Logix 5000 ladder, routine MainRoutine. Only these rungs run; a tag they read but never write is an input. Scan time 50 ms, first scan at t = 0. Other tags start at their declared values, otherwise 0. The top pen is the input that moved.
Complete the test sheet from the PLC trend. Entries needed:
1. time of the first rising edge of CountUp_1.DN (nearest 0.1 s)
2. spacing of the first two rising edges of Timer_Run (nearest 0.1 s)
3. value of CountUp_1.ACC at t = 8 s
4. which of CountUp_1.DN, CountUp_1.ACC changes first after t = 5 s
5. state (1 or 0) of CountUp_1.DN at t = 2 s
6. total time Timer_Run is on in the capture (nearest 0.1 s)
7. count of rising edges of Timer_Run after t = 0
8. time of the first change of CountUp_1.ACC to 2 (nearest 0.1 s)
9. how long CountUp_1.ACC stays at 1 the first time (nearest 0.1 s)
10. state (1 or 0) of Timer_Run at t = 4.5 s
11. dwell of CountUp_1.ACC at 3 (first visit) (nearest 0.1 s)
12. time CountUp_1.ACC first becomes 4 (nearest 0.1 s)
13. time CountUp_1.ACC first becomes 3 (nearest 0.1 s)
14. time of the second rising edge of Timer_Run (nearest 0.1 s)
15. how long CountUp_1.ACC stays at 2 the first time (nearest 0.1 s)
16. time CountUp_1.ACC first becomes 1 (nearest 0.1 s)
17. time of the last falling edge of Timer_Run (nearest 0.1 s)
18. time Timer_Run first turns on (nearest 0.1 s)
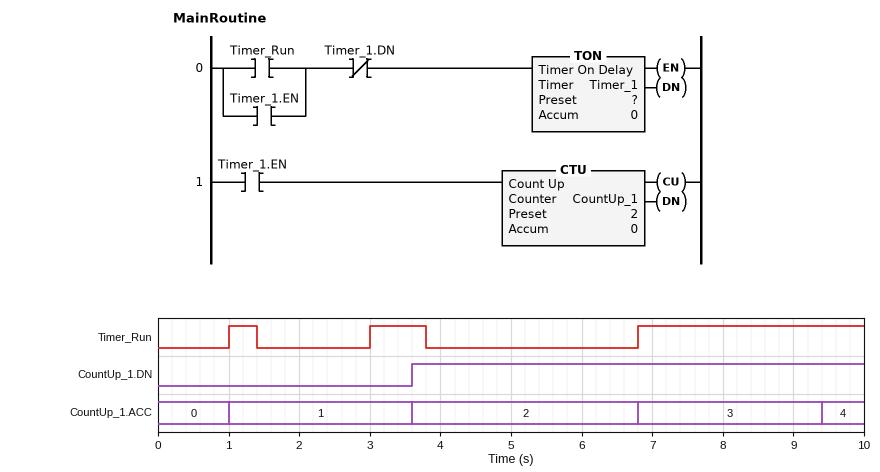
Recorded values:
3.6 s
2.0 s
3
CountUp_1.ACC
0
4.4 s
3
3.6 s
2.6 s
0
2.6 s
9.4 s
6.8 s
3.0 s
3.2 s
1.0 s
3.8 s
1.0 s
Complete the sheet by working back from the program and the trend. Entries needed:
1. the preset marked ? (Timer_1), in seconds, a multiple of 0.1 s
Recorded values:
2.5 s
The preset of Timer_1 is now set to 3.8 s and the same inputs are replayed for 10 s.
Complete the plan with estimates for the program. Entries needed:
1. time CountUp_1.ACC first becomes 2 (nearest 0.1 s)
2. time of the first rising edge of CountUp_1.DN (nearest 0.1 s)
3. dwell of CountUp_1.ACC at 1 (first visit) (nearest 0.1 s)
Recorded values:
6.8 s
6.8 s
5.8 s
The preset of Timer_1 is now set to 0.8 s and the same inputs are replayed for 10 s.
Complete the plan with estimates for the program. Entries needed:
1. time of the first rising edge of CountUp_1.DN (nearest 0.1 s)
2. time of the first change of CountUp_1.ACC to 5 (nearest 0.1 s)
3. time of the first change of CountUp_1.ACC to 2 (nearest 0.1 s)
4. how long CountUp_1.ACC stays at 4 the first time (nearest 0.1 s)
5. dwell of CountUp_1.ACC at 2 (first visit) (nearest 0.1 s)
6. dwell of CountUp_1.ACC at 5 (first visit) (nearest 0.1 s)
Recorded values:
3.0 s
8.6 s
3.0 s
0.9 s
3.8 s
0.9 s
